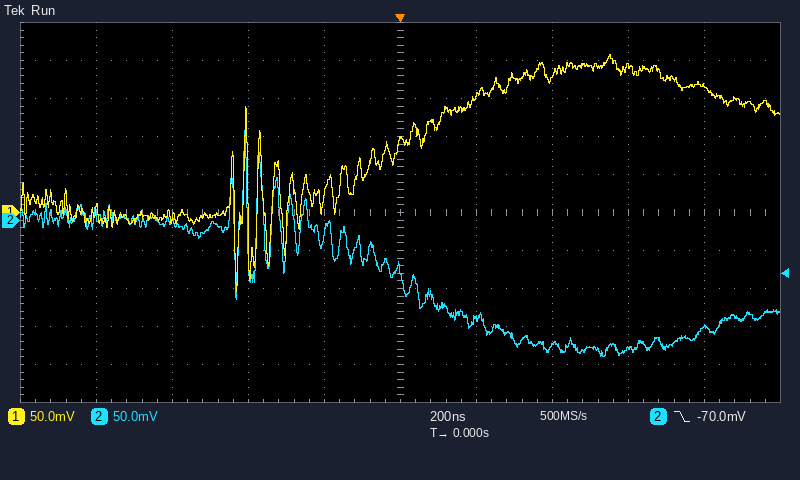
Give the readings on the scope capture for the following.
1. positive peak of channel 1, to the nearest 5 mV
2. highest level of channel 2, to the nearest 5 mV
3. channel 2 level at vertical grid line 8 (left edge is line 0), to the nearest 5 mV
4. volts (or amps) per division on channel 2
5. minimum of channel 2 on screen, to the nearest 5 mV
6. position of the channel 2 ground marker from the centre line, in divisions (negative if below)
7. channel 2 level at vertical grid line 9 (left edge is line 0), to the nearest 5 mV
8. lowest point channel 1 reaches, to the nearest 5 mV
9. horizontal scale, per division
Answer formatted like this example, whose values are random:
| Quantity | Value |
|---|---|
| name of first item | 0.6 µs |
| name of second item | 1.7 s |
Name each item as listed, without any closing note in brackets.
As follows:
| Quantity | Value |
|---|---|
| positive peak of channel 1, to the nearest 5 mV | 210 mV |
| highest level of channel 2, to the nearest 5 mV | 120 mV |
| channel 2 level at vertical grid line 8 (left edge is line 0), to the nearest 5 mV | -170 mV |
| volts (or amps) per division on channel 2 | 50 mV |
| minimum of channel 2 on screen, to the nearest 5 mV | -180 mV |
| position of the channel 2 ground marker from the centre line, in divisions | -0.2 div |
| channel 2 level at vertical grid line 9 (left edge is line 0), to the nearest 5 mV | -140 mV |
| lowest point channel 1 reaches, to the nearest 5 mV | -105 mV |
| horizontal scale, per division | 200 ns |
